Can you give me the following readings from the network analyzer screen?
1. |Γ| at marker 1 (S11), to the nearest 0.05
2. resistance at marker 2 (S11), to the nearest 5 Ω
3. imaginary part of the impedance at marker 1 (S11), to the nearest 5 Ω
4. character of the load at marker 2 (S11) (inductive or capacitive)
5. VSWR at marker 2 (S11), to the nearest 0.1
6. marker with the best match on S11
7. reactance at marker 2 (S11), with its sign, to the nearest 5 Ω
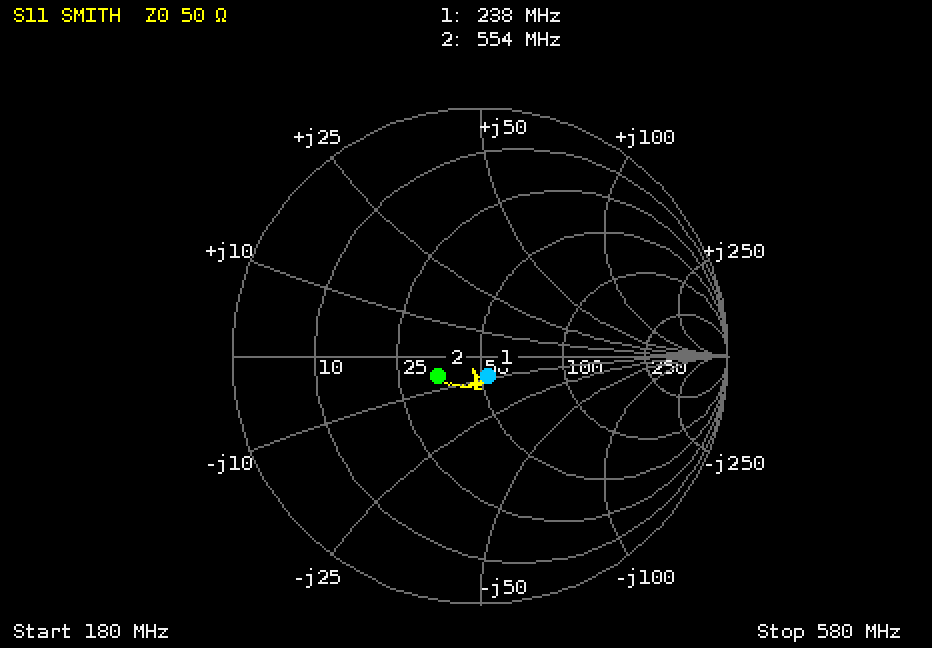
0.10
35 Ω
-10 Ω
capacitive
1.5
marker 1
-5 Ω
